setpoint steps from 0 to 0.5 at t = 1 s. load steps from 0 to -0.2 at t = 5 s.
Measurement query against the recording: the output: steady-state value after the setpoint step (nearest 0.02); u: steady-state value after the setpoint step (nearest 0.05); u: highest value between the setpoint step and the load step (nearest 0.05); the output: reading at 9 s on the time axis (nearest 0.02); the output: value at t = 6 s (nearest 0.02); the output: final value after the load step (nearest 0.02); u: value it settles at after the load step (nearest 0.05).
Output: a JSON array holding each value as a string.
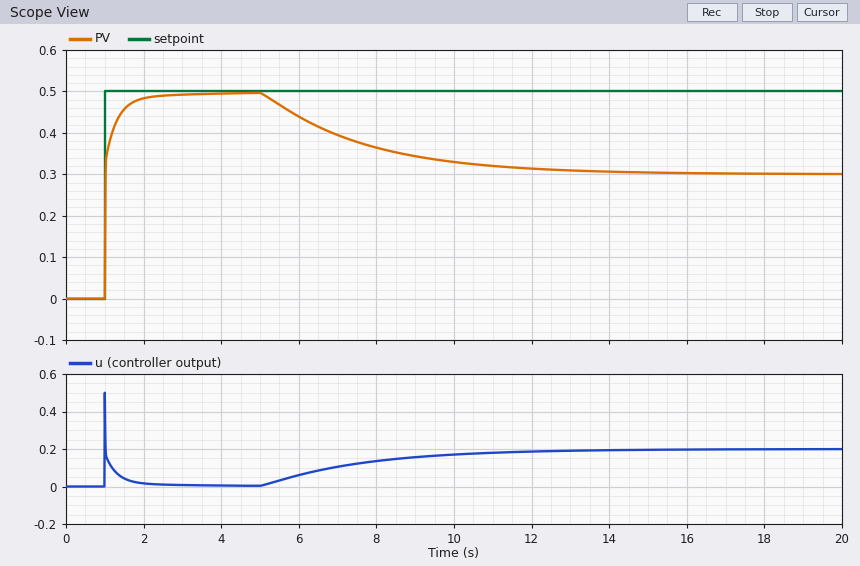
["0.50", "0.00", "0.50", "0.34", "0.44", "0.30", "0.20"]
